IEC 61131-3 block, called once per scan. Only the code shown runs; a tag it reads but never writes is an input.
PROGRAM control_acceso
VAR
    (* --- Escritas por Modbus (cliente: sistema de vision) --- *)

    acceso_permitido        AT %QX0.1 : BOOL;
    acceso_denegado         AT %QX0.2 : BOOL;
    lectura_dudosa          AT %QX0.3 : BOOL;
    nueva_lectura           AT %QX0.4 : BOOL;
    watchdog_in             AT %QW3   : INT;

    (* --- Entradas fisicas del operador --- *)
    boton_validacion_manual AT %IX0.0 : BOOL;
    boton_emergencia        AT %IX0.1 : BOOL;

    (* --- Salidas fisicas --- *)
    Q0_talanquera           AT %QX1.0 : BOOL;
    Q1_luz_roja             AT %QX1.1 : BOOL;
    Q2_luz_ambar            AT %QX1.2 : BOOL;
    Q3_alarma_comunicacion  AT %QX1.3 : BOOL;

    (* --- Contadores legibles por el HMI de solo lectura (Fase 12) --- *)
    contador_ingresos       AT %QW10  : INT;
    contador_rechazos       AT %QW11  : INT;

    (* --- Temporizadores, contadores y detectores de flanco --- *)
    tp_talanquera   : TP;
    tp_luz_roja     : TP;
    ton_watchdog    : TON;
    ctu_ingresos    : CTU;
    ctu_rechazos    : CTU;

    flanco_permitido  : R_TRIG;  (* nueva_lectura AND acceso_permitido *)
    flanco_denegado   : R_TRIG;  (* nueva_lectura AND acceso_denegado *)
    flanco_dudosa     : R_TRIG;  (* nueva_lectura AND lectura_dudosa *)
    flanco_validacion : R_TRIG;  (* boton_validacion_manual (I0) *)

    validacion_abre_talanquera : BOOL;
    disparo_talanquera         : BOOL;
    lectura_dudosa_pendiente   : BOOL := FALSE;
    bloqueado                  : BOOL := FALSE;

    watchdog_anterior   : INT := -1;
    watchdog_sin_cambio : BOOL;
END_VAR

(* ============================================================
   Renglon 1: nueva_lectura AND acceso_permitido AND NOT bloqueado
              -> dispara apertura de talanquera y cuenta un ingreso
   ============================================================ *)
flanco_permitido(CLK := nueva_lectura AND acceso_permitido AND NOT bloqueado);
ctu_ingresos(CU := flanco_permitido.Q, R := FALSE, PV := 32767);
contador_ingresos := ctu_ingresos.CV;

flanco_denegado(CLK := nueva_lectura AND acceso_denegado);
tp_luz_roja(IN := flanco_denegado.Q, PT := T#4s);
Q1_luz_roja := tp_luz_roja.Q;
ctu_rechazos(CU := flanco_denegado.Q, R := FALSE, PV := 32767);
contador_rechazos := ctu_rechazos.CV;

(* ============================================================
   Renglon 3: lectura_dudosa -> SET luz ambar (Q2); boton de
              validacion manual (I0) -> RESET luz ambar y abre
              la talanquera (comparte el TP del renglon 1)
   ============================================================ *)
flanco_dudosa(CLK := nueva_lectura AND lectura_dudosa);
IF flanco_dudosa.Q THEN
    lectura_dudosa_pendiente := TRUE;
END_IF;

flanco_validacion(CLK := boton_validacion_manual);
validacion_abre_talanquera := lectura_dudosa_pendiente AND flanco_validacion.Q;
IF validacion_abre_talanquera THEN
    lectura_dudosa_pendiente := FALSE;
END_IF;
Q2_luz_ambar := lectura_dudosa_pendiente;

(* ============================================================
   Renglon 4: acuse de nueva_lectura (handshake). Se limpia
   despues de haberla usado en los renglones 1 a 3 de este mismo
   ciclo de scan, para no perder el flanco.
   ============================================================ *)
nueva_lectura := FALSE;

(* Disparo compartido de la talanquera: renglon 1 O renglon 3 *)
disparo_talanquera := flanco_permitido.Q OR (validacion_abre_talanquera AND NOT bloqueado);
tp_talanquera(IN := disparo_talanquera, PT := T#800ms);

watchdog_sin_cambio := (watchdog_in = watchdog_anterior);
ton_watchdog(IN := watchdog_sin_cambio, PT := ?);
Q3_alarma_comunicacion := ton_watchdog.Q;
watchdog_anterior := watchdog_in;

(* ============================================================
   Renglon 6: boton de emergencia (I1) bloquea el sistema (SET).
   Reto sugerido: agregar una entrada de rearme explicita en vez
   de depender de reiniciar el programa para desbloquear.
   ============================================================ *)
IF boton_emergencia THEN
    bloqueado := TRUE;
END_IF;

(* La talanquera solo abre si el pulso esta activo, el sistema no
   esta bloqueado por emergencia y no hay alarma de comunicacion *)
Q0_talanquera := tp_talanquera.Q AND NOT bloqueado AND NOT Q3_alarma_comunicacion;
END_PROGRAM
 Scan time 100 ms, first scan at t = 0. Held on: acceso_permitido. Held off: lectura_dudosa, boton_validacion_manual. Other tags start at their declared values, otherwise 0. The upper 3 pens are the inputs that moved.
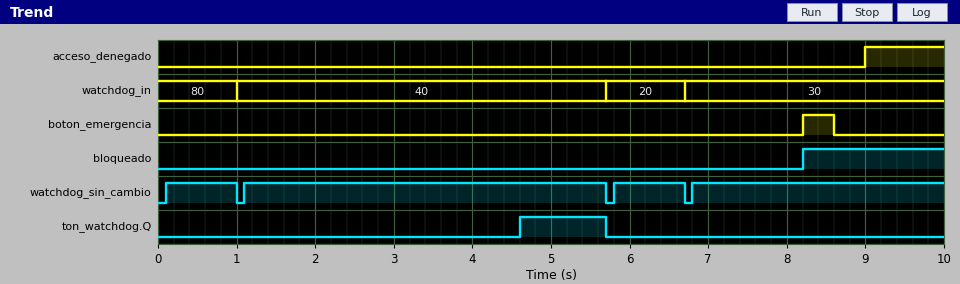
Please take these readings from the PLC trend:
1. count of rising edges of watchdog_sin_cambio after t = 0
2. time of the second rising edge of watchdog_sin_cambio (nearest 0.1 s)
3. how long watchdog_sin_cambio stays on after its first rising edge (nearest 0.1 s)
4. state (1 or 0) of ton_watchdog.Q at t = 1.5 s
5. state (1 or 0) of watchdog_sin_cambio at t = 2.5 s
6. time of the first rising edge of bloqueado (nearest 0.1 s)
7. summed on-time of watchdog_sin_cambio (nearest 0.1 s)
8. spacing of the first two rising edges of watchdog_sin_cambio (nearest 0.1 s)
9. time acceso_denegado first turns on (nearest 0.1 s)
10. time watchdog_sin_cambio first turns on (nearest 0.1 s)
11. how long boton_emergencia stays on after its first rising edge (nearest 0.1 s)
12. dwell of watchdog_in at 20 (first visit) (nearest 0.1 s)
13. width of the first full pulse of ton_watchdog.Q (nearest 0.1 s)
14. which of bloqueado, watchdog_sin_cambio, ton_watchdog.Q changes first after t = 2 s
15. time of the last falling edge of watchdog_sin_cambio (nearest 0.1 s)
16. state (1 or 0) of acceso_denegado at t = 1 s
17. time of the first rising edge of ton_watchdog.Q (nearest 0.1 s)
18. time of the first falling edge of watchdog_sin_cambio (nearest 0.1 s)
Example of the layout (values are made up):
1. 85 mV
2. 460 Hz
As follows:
1. 4
2. 1.1 s
3. 0.9 s
4. 0
5. 1
6. 8.2 s
7. 9.6 s
8. 1.0 s
9. 9.0 s
10. 0.1 s
11. 0.4 s
12. 1.0 s
13. 1.1 s
14. ton_watchdog.Q
15. 6.7 s
16. 0
17. 4.6 s
18. 1.0 s
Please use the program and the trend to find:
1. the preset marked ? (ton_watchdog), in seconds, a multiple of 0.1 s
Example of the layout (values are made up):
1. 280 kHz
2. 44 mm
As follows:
1. 3.5 s
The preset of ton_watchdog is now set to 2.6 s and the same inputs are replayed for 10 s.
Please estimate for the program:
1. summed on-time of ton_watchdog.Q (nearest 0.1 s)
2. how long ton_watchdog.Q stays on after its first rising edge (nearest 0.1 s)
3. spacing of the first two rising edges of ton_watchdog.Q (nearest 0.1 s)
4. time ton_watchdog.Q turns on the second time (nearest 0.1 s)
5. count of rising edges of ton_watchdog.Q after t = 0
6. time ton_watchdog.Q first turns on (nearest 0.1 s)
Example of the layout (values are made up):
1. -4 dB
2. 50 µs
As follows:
1. 2.6 s
2. 2.0 s
3. 5.7 s
4. 9.4 s
5. 2
6. 3.7 s
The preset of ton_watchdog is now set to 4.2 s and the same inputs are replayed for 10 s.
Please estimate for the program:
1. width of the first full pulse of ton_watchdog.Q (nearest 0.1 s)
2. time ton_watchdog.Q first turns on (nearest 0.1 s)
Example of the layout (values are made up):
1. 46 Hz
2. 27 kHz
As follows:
1. 0.4 s
2. 5.3 s
